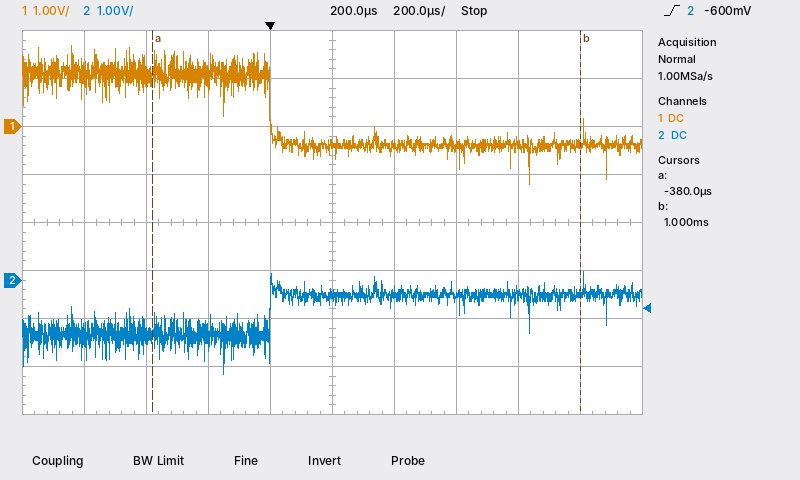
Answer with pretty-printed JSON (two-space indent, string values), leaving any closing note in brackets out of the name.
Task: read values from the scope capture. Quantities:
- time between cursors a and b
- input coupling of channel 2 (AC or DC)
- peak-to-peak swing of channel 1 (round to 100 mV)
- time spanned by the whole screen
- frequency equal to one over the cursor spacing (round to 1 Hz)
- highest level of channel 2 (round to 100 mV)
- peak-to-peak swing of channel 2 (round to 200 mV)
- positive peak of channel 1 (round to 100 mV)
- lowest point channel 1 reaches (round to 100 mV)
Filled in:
{
  "time between cursors a and b": "1.38 ms",
  "input coupling of channel 2": "DC",
  "peak-to-peak swing of channel 1": "2.9 V",
  "time spanned by the whole screen": "2 ms",
  "frequency equal to one over the cursor spacing": "725 Hz",
  "highest level of channel 2": "200 mV",
  "peak-to-peak swing of channel 2": "2.2 V",
  "positive peak of channel 1": "1.7 V",
  "lowest point channel 1 reaches": "-1.2 V"
}
